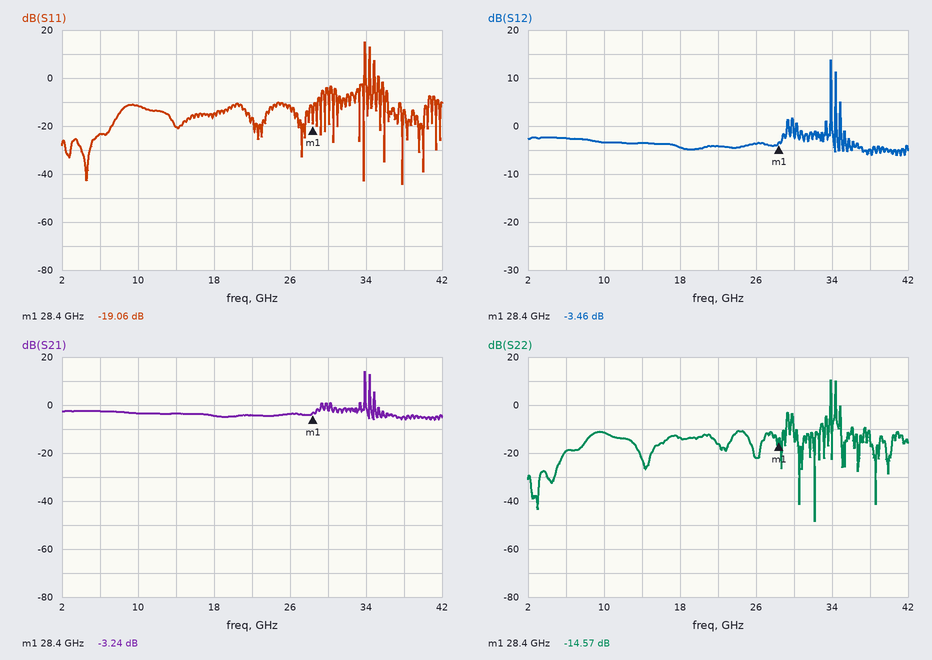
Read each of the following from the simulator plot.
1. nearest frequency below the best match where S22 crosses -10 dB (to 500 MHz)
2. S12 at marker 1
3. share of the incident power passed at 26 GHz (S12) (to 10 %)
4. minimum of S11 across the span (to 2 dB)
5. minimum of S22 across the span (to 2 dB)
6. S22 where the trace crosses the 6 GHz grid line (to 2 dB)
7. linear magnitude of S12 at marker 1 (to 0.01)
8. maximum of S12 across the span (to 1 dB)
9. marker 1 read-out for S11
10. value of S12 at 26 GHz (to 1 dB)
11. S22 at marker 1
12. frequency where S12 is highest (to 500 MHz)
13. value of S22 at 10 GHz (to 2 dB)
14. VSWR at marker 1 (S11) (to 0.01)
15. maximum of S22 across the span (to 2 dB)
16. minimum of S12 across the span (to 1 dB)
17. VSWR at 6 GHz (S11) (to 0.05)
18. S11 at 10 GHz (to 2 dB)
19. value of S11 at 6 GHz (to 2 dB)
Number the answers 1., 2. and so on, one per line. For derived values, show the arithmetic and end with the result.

1. 30.0 GHz
2. -3.46 dB
3. 10^(-4/10) ≈ 40 %
4. -44 dB
5. -48 dB
6. -20 dB
7. 10^(-3.46/20) ≈ 0.67
8. 14 dB
9. -19.06 dB
10. -4 dB
11. -14.57 dB
12. 34.0 GHz
13. -12 dB
14. (1 + 0.1114)/(1 − 0.1114) ≈ 1.25
15. 10 dB
16. -6 dB
17. |Γ| = 10^(-24/20) = 0.0631; VSWR = (1 + 0.0631)/(1 − 0.0631) ≈ 1.13, so 1.15 to the nearest 0.05
18. -12 dB
19. -24 dB
